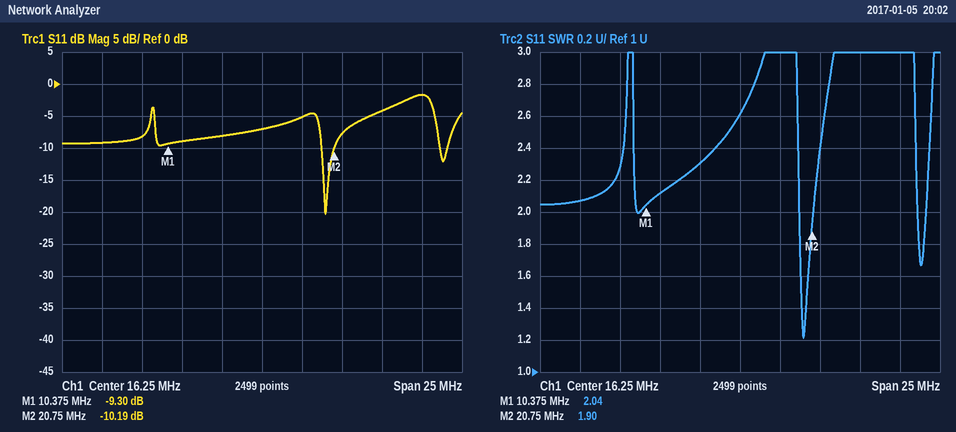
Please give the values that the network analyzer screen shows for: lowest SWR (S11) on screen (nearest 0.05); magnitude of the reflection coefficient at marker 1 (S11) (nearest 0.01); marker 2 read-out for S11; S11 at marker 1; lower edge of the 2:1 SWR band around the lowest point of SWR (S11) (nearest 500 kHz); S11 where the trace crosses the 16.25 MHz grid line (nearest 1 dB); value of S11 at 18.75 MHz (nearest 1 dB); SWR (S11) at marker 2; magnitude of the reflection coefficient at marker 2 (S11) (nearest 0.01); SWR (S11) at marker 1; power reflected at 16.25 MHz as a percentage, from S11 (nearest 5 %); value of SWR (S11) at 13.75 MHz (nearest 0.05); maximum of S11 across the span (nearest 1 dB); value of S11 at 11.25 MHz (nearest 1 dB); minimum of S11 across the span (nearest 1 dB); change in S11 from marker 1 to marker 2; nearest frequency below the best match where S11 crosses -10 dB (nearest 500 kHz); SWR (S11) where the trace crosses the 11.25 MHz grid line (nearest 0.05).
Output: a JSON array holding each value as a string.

["1.20", "0.34", "-10.19 dB", "-9.30 dB", "20.0 MHz", "-7 dB", "-5 dB", "1.90", "0.31", "2.04", "20 %", "2.30", "-2 dB", "-9 dB", "-20 dB", "-0.89 dB", "20.0 MHz", "2.10"]
